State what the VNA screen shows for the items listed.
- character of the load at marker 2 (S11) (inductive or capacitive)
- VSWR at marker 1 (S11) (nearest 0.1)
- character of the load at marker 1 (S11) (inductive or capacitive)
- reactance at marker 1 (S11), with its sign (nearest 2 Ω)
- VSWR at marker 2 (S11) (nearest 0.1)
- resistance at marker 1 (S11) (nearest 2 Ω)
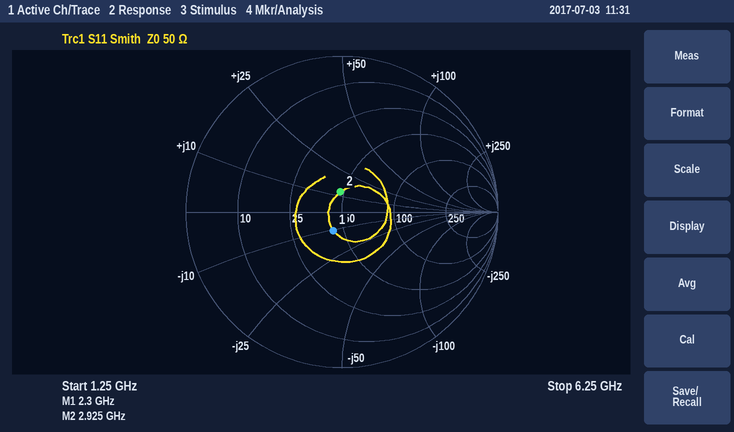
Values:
inductive
1.3
capacitive
-10 Ω
1.3
44 Ω
